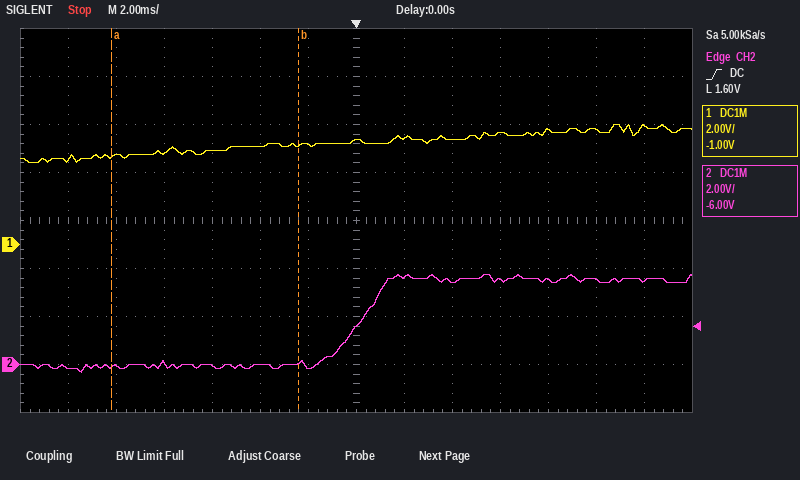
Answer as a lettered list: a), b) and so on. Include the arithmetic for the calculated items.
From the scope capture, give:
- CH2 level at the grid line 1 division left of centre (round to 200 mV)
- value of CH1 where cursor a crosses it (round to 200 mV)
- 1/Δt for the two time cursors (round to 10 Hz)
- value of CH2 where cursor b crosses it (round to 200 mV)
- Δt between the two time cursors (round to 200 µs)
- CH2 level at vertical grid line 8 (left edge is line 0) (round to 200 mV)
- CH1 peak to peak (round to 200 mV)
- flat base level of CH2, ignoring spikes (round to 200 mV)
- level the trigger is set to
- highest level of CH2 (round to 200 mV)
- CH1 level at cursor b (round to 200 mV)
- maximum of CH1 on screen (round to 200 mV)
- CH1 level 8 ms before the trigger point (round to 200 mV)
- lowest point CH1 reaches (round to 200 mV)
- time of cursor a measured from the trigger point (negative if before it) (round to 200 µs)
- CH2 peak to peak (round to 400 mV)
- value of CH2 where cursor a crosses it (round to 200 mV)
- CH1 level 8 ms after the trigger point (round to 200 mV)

a) -200 mV
b) 3.6 V
c) 1 / 7.8 ms ≈ 130 Hz
d) 0.0 V
e) 7.8 ms
f) 3.6 V
g) 5.0 V − (3.4 V) = 1.6 V
h) 0.0 V
i) 1.60 V
j) 3.8 V
k) 4.2 V
l) 5.0 V
m) 3.8 V
n) 3.4 V
o) -10.2 ms
p) 4.0 V
q) 0.0 V
r) 4.8 V
